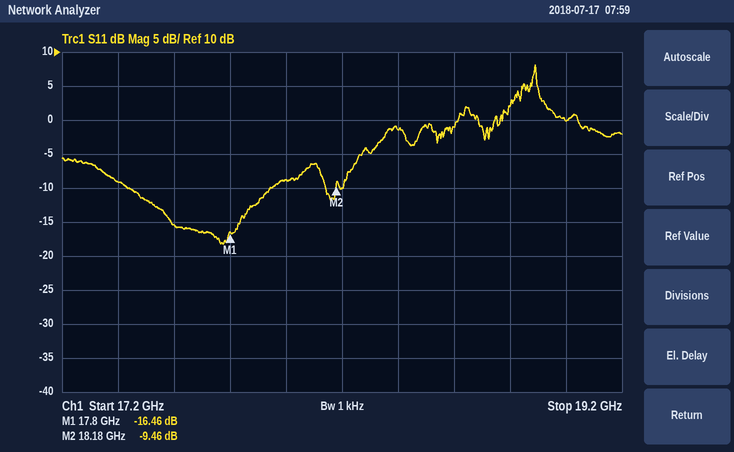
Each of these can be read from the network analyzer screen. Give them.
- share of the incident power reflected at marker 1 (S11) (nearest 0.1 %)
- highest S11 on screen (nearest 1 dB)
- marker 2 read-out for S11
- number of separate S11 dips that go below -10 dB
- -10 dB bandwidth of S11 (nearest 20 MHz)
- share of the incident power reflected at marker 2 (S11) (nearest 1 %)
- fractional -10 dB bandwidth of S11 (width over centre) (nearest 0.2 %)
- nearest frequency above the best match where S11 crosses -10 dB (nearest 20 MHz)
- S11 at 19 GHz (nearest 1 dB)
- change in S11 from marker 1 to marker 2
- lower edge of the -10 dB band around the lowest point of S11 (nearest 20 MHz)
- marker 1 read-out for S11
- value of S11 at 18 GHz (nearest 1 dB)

2.3 %
8 dB
-9.46 dB
2
500 MHz
11 %
2.8 %
17.94 GHz
0 dB
7.00 dB
17.44 GHz
-16.46 dB
-9 dB
